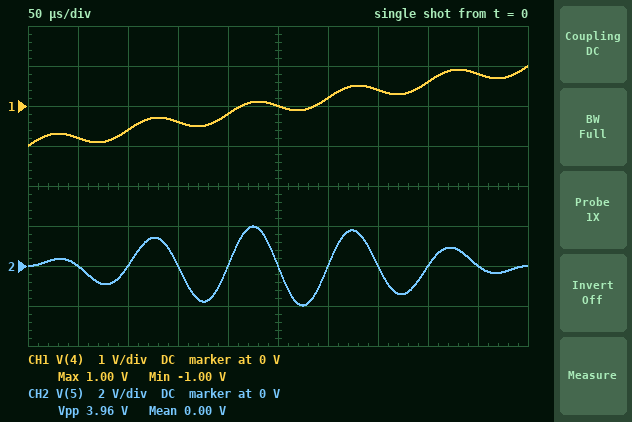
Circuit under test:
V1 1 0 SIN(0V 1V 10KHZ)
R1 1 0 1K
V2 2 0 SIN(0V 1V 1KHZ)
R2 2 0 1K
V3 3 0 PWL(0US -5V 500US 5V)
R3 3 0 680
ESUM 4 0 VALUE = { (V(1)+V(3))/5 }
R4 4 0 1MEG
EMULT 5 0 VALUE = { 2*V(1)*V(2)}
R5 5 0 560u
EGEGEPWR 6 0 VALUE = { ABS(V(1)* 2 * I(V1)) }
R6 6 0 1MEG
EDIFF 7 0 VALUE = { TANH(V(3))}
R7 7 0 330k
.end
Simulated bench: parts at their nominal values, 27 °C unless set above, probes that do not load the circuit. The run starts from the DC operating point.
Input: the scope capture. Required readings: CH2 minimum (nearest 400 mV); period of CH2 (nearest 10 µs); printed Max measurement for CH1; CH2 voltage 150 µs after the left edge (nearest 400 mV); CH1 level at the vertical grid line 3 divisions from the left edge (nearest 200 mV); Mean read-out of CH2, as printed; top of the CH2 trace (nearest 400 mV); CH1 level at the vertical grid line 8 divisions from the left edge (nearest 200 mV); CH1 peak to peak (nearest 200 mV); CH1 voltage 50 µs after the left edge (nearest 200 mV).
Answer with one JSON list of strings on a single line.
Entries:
["-2.0 V", "100 µs", "1.00 V", "0 V", "-400 mV", "0.00 V", "2.0 V", "600 mV", "2.0 V", "-800 mV"]
